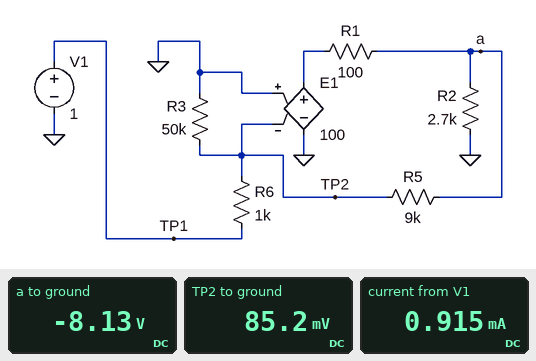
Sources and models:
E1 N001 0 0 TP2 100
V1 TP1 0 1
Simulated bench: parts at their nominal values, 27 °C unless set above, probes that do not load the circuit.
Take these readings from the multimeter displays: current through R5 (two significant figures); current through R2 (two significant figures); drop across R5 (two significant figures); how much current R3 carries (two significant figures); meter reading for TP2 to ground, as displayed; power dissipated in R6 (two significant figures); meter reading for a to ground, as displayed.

910 µA
3.0 mA
8.2 V
1.7 µA
85.2 mV
840 µW
-8.13 V
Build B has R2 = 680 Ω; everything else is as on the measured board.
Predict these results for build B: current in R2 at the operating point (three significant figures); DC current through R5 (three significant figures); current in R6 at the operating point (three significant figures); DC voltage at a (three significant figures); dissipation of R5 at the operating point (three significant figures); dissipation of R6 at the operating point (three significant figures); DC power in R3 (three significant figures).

11.8 mA
905 µA
907 µA
-8.05 V
7.37 mW
822 µW
174 nW
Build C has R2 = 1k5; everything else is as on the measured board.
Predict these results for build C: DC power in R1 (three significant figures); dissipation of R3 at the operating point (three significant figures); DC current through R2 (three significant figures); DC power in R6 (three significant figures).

3.99 mW
153 nW
5.41 mA
833 µW
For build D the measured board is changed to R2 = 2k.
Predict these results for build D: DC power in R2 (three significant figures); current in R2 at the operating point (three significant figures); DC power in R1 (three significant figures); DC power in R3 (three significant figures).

33.0 mW
4.06 mA
2.47 mW
149 nW
